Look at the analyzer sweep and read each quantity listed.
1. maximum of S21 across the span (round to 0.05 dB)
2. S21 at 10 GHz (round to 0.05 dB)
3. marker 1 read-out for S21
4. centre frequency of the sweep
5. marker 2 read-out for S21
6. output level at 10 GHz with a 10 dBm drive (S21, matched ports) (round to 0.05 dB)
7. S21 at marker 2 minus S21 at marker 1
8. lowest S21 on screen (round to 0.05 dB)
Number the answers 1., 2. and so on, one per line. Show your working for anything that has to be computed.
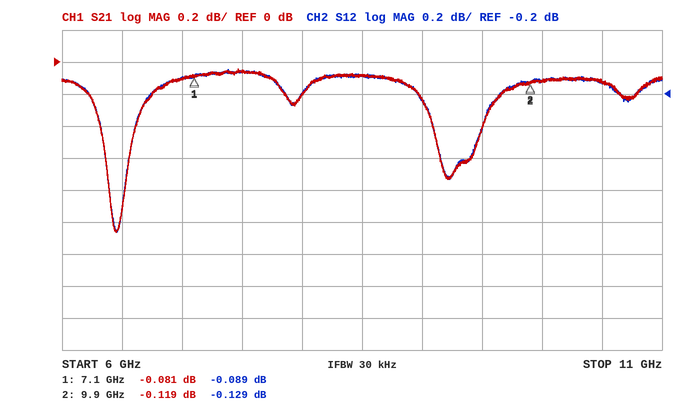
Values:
1. -0.05 dB
2. -0.10 dB
3. -0.081 dB
4. 8.5 GHz
5. -0.119 dB
6. 10 dBm + (-0.10 dB) = 9.90 dBm
7. -0.119 − (-0.081) = -0.038 dB
8. -1.05 dB
